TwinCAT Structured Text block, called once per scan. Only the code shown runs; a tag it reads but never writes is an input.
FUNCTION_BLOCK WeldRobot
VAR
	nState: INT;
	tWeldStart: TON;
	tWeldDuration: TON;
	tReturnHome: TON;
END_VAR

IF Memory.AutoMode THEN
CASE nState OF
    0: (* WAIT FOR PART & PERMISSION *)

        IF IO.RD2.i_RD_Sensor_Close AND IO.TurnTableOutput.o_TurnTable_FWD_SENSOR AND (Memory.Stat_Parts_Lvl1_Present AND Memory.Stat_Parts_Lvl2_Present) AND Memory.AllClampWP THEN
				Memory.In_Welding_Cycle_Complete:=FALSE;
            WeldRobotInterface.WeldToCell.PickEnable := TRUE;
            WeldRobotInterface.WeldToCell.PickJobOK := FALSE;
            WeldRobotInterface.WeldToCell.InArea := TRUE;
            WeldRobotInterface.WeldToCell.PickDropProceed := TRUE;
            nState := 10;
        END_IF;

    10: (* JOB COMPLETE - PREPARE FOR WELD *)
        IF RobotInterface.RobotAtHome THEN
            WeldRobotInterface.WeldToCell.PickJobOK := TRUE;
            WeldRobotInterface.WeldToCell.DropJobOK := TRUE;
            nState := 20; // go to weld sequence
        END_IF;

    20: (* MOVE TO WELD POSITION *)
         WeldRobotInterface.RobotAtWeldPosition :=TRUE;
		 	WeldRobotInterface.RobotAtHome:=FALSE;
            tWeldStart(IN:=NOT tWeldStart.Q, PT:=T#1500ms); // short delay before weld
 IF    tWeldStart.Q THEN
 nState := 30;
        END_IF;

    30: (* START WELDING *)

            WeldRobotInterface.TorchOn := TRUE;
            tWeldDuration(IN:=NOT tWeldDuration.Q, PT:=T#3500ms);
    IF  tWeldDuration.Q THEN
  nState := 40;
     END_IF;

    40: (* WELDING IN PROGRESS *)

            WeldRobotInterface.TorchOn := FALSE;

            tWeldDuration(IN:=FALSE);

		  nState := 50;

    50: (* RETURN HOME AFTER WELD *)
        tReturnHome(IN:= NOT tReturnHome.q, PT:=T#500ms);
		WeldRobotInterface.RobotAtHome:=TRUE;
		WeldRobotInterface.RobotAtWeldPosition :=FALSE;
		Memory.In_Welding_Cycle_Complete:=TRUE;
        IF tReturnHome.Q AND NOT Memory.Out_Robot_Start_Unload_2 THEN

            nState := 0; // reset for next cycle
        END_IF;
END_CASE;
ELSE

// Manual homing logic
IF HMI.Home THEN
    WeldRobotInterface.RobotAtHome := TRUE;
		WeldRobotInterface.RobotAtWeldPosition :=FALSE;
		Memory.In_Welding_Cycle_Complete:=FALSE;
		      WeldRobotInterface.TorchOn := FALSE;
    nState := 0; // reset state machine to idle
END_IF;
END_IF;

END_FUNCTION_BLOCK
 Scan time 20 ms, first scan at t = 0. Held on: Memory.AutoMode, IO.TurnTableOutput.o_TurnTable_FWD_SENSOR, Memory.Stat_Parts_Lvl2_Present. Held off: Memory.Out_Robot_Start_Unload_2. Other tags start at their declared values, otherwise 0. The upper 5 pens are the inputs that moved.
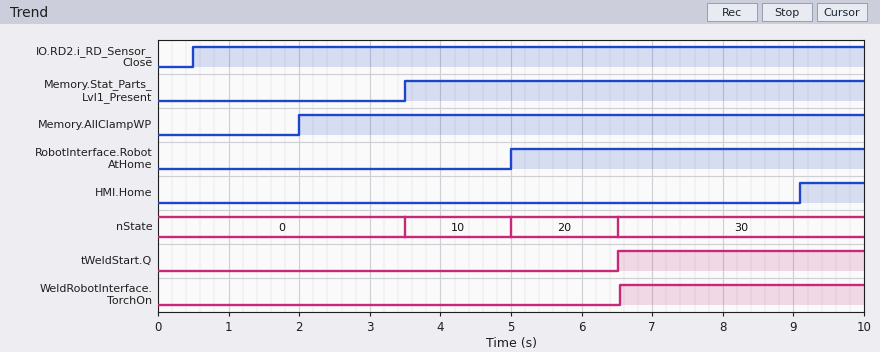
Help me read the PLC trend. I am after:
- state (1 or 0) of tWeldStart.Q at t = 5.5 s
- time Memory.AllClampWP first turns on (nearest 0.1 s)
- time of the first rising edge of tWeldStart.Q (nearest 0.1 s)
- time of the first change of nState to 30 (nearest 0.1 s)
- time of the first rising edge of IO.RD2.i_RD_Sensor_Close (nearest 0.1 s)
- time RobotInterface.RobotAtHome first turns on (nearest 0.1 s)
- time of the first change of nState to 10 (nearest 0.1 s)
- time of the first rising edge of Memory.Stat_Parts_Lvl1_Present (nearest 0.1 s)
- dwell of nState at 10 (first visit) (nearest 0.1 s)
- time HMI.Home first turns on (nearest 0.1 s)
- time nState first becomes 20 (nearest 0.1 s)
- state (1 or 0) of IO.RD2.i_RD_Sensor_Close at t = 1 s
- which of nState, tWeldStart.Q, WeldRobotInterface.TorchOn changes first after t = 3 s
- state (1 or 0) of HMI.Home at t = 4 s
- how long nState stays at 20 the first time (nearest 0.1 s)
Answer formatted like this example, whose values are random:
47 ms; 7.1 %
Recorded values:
0; 2.0 s; 6.5 s; 6.5 s; 0.5 s; 5.0 s; 3.5 s; 3.5 s; 1.5 s; 9.1 s; 5.0 s; 1; nState; 0; 1.5 s
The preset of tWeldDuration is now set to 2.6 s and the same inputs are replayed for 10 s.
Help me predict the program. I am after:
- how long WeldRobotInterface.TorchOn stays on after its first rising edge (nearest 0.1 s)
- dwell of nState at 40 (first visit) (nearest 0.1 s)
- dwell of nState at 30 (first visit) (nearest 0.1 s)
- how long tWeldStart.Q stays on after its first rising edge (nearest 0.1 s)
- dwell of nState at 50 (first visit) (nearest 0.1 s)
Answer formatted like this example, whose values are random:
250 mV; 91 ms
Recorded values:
2.6 s; 0.0 s; 2.6 s; 3.2 s; 0.5 s
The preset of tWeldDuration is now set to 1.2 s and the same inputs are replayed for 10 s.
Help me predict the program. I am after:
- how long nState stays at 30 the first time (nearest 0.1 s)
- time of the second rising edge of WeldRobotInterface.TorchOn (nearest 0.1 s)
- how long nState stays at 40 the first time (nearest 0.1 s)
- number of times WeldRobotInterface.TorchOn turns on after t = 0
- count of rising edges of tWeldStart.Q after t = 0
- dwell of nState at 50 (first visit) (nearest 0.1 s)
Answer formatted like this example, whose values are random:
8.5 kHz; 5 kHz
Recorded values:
1.2 s; 9.9 s; 0.0 s; 2; 2; 0.5 s
